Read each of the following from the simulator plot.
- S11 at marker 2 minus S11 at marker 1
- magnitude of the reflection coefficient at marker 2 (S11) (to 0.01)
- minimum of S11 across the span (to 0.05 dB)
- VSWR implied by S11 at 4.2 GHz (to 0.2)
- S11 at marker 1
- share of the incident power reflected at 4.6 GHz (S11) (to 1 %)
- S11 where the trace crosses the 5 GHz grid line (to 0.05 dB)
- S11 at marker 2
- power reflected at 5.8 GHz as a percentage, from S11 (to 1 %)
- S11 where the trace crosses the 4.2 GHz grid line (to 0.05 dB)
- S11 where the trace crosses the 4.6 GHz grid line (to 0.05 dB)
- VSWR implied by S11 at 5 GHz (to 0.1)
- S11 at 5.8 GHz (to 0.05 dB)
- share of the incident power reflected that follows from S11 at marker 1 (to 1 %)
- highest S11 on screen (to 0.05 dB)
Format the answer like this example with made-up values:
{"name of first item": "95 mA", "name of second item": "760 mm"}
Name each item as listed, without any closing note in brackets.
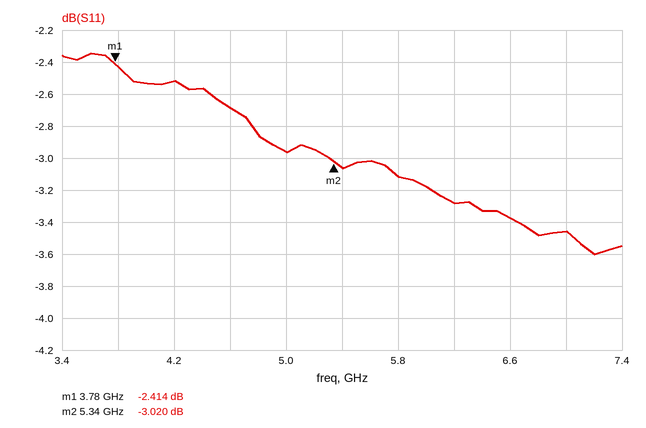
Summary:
{"S11 at marker 2 minus S11 at marker 1": "-0.606 dB", "magnitude of the reflection coefficient at marker 2 (S11)": "0.71", "minimum of S11 across the span": "-3.60 dB", "VSWR implied by S11 at 4.2 GHz": "7.0", "S11 at marker 1": "-2.414 dB", "share of the incident power reflected at 4.6 GHz (S11)": "54 %", "S11 where the trace crosses the 5 GHz grid line": "-2.95 dB", "S11 at marker 2": "-3.020 dB", "power reflected at 5.8 GHz as a percentage, from S11": "49 %", "S11 where the trace crosses the 4.2 GHz grid line": "-2.50 dB", "S11 where the trace crosses the 4.6 GHz grid line": "-2.70 dB", "VSWR implied by S11 at 5 GHz": "5.9", "S11 at 5.8 GHz": "-3.10 dB", "share of the incident power reflected that follows from S11 at marker 1": "57 %", "highest S11 on screen": "-2.35 dB"}
